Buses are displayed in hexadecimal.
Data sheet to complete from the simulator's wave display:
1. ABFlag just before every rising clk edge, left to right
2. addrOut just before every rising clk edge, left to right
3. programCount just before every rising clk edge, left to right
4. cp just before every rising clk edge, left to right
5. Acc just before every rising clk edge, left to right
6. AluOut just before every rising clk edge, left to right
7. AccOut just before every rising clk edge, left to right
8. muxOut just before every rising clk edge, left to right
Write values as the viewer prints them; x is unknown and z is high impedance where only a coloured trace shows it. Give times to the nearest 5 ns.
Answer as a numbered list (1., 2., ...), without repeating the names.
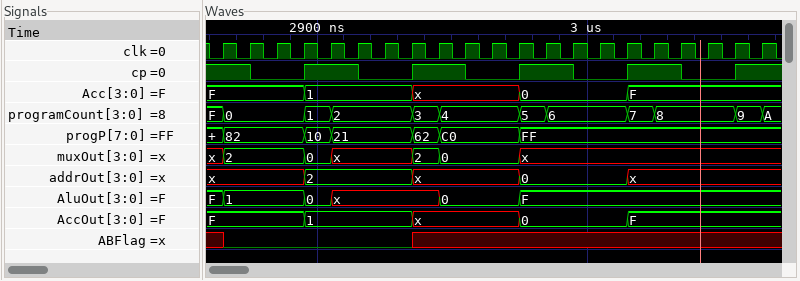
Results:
1. x 0 0 0 0 0 0 0 x x x x x x x x x x x x x
2. x, x, x, x, 2, 2, 2, 2, x, x, x, x, 0, 0, 0, 0, x, x, x, x, x
3. F, 0, 0, 0, 1, 2, 2, 2, 3, 4, 4, 4, 5, 6, 6, 6, 7, 8, 8, 8, 9
4. 1 1 0 0 1 1 0 0 1 1 0 0 1 1 0 0 1 1 0 0 1
5. F, F, F, F, 1, 1, 1, 1, x, x, x, x, 0, 0, 0, 0, F, F, F, F, F
6. F, 1, 1, 1, 0, x, x, x, x, 0, 0, 0, F, F, F, F, F, F, F, F, F
7. F, F, F, F, 1, 1, 1, 1, x, x, x, x, 0, 0, 0, 0, F, F, F, F, F
8. x, 2, 2, 2, 0, x, x, x, 2, 0, 0, 0, x, x, x, x, x, x, x, x, x
